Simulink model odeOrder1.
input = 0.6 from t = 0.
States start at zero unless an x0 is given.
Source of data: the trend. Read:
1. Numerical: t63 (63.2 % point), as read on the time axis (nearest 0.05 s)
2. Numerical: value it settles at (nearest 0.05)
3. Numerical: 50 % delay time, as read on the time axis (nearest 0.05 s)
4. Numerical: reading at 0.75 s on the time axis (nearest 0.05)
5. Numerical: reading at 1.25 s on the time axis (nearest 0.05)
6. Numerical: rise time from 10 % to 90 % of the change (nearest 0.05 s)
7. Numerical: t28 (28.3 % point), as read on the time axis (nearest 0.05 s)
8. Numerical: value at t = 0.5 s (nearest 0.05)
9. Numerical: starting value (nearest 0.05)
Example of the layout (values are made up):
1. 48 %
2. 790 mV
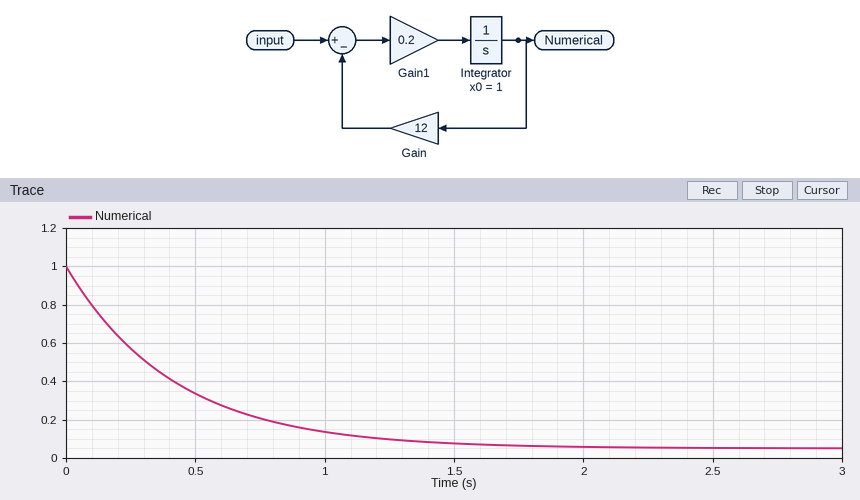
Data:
1. 0.40 s
2. 0.05
3. 0.30 s
4. 0.20
5. 0.10
6. 0.90 s
7. 0.15 s
8. 0.35
9. 1.00
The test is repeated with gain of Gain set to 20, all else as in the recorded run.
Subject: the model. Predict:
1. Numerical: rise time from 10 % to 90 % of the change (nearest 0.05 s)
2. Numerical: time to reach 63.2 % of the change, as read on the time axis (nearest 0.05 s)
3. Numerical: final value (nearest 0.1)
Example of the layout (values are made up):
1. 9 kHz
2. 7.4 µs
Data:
1. 0.55 s
2. 0.25 s
3. 0.0
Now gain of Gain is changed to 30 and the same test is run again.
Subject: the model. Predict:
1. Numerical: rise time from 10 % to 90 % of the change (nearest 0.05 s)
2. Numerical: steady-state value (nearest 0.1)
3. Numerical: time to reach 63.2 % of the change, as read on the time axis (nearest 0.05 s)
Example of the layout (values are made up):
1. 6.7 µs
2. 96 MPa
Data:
1. 0.35 s
2. 0.0
3. 0.15 s
